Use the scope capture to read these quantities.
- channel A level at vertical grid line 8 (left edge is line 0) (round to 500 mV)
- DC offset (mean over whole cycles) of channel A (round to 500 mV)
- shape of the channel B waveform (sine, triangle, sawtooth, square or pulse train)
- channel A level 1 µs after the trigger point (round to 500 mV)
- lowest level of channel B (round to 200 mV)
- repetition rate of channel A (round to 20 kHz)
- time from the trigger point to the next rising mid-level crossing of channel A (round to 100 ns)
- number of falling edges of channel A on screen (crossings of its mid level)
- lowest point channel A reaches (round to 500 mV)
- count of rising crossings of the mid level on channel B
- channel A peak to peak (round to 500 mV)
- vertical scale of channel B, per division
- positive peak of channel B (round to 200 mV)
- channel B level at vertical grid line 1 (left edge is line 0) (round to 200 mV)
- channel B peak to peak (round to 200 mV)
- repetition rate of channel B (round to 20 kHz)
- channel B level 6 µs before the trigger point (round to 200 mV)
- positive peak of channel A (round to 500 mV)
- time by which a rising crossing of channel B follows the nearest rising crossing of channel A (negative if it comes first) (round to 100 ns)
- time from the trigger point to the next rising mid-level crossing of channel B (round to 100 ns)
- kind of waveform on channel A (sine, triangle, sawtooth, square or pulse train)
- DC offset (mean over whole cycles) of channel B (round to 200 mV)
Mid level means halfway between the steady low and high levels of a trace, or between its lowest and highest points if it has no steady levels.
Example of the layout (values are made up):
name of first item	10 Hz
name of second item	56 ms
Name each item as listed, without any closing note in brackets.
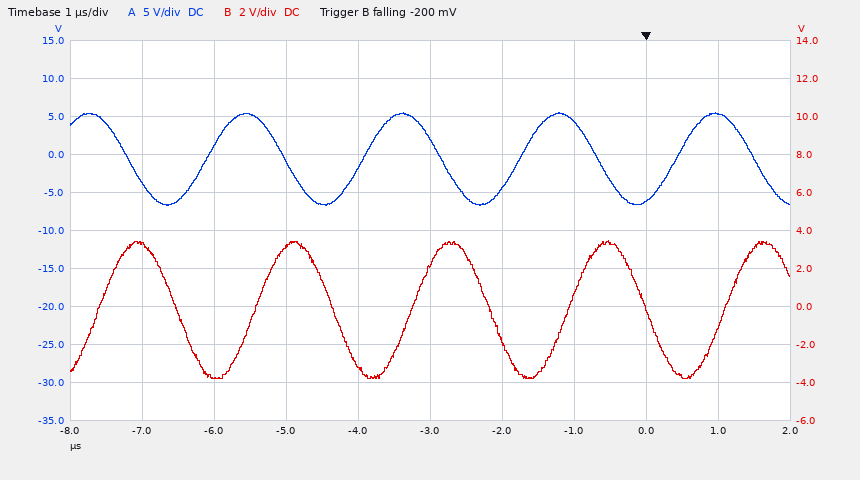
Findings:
channel A level at vertical grid line 8 (left edge is line 0)	-6.0 V
DC offset (mean over whole cycles) of channel A	-500 mV
shape of the channel B waveform	sine
channel A level 1 µs after the trigger point	5.5 V
lowest level of channel B	-3.8 V
repetition rate of channel A	460 kHz
time from the trigger point to the next rising mid-level crossing of channel A	400 ns
number of falling edges of channel A on screen	5
lowest point channel A reaches	-6.5 V
count of rising crossings of the mid level on channel B	5
channel A peak to peak	12.0 V
vertical scale of channel B, per division	2 V
positive peak of channel B	3.4 V
channel B level at vertical grid line 1 (left edge is line 0)	3.2 V
channel B peak to peak	7.2 V
repetition rate of channel B	460 kHz
channel B level 6 µs before the trigger point	-3.8 V
positive peak of channel A	5.5 V
time by which a rising crossing of channel B follows the nearest rising crossing of channel A (negative if it comes first)	+700 ns
time from the trigger point to the next rising mid-level crossing of channel B	1.1 µs
kind of waveform on channel A	sine
DC offset (mean over whole cycles) of channel B	-200 mV
